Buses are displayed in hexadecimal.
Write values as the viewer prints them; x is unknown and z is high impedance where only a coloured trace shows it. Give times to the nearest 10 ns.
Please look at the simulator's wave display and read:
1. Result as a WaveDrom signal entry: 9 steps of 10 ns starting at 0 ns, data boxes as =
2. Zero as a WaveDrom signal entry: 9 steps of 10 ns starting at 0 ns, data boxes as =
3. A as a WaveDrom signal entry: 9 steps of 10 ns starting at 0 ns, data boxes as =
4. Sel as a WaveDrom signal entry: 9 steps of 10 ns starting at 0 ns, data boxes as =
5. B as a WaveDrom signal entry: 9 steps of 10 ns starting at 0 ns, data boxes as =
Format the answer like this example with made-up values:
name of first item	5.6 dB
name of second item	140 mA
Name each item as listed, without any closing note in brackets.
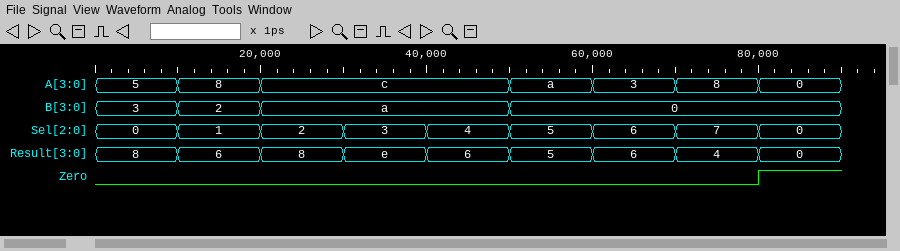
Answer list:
Result as a WaveDrom signal entry: 9 steps of 10 ns starting at 0 ns, data boxes as =	{name: 'Result', wave: '=========', data: '8 6 8 e 6 5 6 4 0'}
Zero as a WaveDrom signal entry: 9 steps of 10 ns starting at 0 ns, data boxes as =	{name: 'Zero', wave: '0.......1'}
A as a WaveDrom signal entry: 9 steps of 10 ns starting at 0 ns, data boxes as =	{name: 'A', wave: '===..====', data: '5 8 c a 3 8 0'}
Sel as a WaveDrom signal entry: 9 steps of 10 ns starting at 0 ns, data boxes as =	{name: 'Sel', wave: '=========', data: '0 1 2 3 4 5 6 7 0'}
B as a WaveDrom signal entry: 9 steps of 10 ns starting at 0 ns, data boxes as =	{name: 'B', wave: '===..=...', data: '3 2 a 0'}
